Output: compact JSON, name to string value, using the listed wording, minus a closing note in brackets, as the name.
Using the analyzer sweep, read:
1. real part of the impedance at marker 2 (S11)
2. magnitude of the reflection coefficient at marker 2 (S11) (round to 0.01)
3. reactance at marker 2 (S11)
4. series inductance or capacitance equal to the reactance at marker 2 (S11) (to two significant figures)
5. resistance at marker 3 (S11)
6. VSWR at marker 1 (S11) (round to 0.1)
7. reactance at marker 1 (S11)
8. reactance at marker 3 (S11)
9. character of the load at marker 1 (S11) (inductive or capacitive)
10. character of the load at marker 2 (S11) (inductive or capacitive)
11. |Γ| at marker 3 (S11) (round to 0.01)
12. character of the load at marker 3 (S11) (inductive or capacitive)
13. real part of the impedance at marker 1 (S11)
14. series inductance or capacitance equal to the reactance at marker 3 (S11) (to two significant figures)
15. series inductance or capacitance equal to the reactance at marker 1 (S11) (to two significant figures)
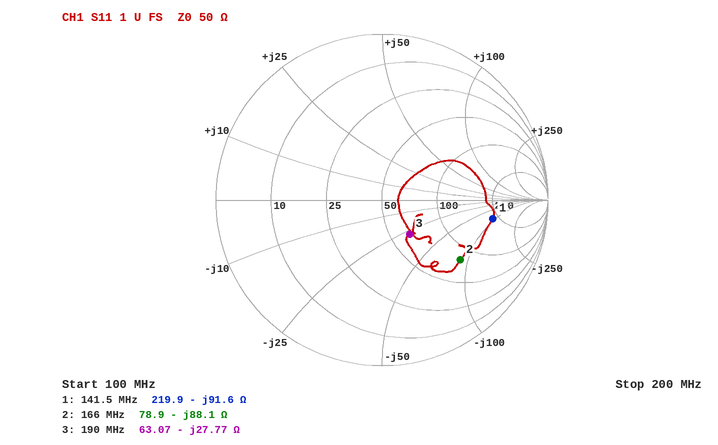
{"real part of the impedance at marker 2": "78.9 Ω", "magnitude of the reflection coefficient at marker 2 (S11)": "0.59", "reactance at marker 2": "-88.1 Ω", "series inductance or capacitance equal to the reactance at marker 2 (S11)": "11 pF", "resistance at marker 3": "63.07 Ω", "VSWR at marker 1 (S11)": "5.2", "reactance at marker 1": "-91.6 Ω", "reactance at marker 3": "-27.77 Ω", "character of the load at marker 1 (S11)": "capacitive", "character of the load at marker 2 (S11)": "capacitive", "|Γ| at marker 3 (S11)": "0.26", "character of the load at marker 3 (S11)": "capacitive", "real part of the impedance at marker 1": "219.9 Ω", "series inductance or capacitance equal to the reactance at marker 3 (S11)": "30 pF", "series inductance or capacitance equal to the reactance at marker 1 (S11)": "12 pF"}
